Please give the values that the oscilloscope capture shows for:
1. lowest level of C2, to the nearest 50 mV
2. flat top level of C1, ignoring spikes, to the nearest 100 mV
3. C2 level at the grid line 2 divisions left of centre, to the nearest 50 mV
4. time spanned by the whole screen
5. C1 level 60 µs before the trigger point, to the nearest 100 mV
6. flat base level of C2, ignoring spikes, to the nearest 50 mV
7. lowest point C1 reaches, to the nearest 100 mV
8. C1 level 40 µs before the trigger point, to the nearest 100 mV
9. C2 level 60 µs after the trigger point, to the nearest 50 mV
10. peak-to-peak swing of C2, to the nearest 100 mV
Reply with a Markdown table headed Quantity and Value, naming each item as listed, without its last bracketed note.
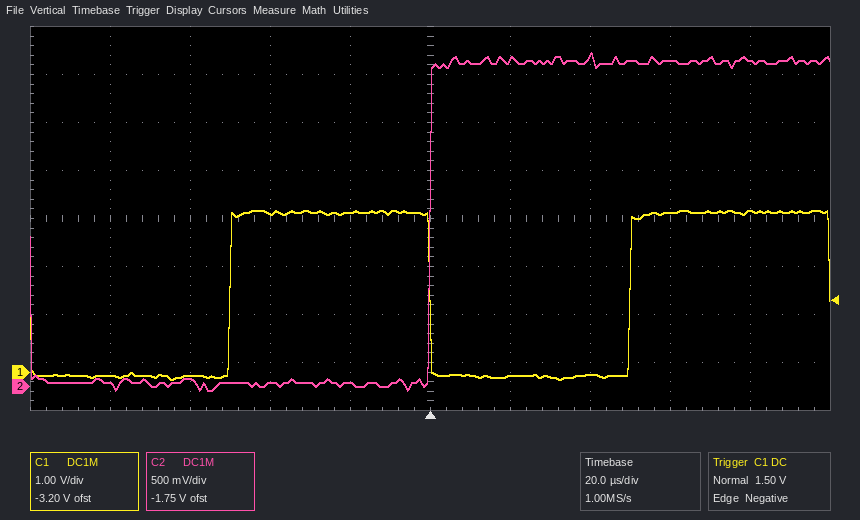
| Quantity | Value |
|---|---|
| lowest level of C2, to the nearest 50 mV | -50 mV |
| flat top level of C1, ignoring spikes, to the nearest 100 mV | 3.3 V |
| C2 level at the grid line 2 divisions left of centre, to the nearest 50 mV | 50 mV |
| time spanned by the whole screen | 200 µs |
| C1 level 60 µs before the trigger point, to the nearest 100 mV | -100 mV |
| flat base level of C2, ignoring spikes, to the nearest 50 mV | 50 mV |
| lowest point C1 reaches, to the nearest 100 mV | -200 mV |
| C1 level 40 µs before the trigger point, to the nearest 100 mV | 3.3 V |
| C2 level 60 µs after the trigger point, to the nearest 50 mV | 3.40 V |
| peak-to-peak swing of C2, to the nearest 100 mV | 3.50 V |
